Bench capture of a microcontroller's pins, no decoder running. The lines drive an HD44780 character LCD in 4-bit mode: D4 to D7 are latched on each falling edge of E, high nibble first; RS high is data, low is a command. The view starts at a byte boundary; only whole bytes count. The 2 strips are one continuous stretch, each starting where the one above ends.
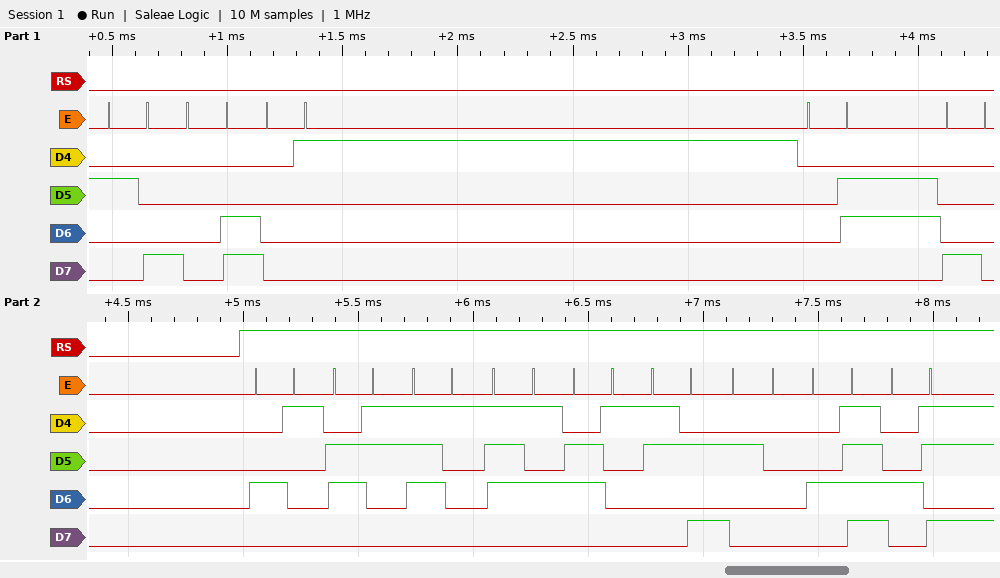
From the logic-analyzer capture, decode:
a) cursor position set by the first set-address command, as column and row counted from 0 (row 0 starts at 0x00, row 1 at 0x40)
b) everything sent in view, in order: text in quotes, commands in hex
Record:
column 0, row 0
0x28 0x0C 0x01 0x06 0x80 "Acqua: OK"
